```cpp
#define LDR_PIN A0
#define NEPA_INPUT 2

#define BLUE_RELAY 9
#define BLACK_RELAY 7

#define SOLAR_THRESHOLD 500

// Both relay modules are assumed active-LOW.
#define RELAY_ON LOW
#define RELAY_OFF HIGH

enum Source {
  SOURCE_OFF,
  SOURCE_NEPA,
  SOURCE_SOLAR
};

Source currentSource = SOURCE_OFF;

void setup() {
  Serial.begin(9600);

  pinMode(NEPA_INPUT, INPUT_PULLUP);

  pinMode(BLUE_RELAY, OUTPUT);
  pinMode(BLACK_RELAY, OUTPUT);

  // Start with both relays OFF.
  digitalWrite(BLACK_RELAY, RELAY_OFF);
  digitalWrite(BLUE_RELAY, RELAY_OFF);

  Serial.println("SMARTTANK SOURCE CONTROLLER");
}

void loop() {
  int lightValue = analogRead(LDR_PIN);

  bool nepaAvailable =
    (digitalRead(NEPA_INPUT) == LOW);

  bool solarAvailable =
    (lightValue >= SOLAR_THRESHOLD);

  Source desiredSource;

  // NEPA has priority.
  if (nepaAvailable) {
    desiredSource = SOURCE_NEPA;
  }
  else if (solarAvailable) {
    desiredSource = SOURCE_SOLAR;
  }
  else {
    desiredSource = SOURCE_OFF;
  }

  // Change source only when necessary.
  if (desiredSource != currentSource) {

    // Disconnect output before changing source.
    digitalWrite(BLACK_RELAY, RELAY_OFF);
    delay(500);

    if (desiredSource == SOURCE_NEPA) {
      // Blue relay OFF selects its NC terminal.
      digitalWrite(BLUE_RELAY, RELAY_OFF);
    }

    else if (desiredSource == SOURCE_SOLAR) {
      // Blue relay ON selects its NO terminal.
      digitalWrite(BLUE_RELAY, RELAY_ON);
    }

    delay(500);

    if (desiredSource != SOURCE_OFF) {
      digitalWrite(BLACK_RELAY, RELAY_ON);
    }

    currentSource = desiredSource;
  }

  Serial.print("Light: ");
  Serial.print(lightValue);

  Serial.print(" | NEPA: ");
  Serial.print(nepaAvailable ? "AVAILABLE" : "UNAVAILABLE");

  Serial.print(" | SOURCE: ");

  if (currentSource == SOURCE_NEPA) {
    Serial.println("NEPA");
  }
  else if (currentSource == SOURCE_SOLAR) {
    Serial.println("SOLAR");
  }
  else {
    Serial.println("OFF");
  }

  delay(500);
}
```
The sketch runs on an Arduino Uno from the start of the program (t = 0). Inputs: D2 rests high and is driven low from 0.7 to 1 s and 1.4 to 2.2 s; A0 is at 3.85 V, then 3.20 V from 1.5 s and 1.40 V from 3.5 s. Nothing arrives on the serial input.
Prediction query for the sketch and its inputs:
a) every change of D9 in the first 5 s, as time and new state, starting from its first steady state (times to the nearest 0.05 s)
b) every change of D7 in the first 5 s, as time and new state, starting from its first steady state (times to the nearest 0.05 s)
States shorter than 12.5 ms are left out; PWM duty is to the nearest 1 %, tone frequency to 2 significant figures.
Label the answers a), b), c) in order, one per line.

a) 0 s high; 0.5 s low; 2 s high; 3.5 s low
b) 0 s high; 1 s low; 1.5 s high; 2.5 s low; 3 s high; 4 s low; 4.5 s high
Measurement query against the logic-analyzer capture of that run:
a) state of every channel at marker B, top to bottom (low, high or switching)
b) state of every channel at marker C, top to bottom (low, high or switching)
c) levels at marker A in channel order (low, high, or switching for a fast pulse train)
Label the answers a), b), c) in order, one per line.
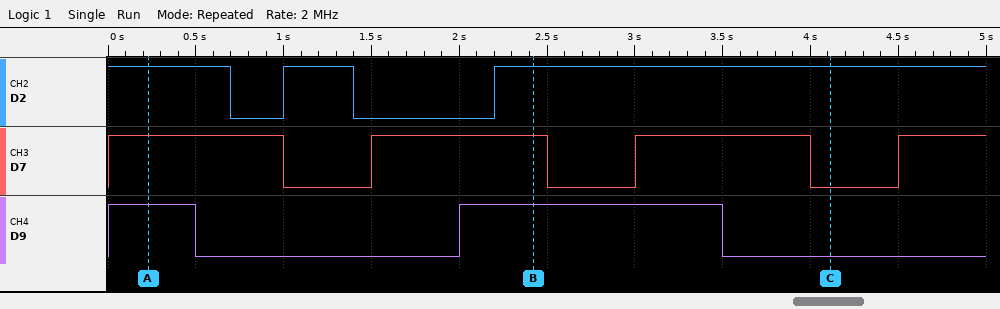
a) D2 high, D7 high, D9 high
b) D2 high, D7 low, D9 low
c) D2 high, D7 high, D9 high
